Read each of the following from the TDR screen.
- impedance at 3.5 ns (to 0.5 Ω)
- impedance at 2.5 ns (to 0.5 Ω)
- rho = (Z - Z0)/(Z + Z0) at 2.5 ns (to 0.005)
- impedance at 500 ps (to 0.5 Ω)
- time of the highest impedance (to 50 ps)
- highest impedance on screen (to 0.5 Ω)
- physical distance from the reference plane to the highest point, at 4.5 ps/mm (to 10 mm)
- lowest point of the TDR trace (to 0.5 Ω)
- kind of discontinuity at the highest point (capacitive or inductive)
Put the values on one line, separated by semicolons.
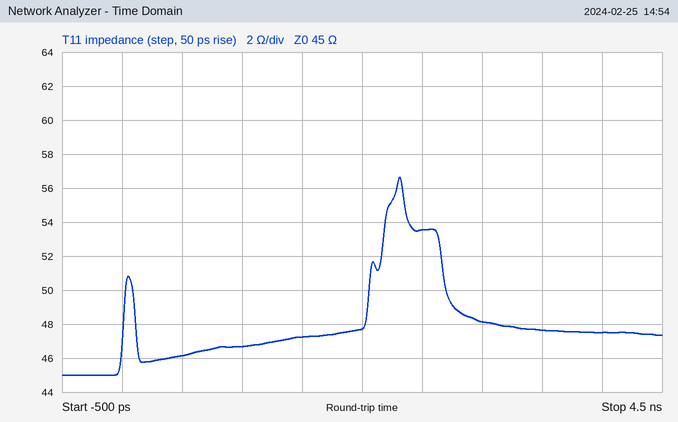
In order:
47.5 Ω; 53.5 Ω; +0.085; 46.0 Ω; 2.30 ns; 56.5 Ω; 260 mm; 45.0 Ω; inductive
